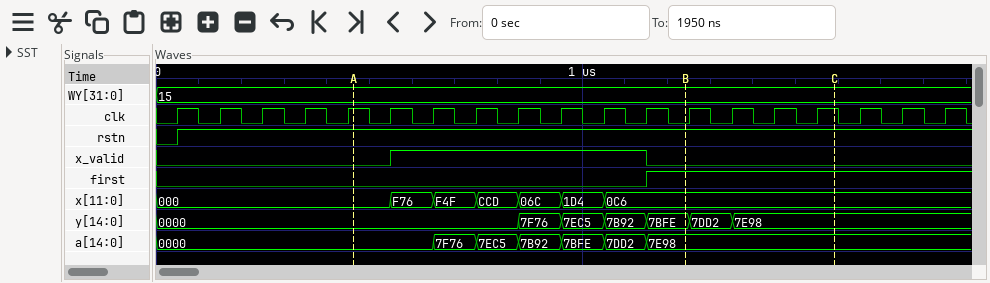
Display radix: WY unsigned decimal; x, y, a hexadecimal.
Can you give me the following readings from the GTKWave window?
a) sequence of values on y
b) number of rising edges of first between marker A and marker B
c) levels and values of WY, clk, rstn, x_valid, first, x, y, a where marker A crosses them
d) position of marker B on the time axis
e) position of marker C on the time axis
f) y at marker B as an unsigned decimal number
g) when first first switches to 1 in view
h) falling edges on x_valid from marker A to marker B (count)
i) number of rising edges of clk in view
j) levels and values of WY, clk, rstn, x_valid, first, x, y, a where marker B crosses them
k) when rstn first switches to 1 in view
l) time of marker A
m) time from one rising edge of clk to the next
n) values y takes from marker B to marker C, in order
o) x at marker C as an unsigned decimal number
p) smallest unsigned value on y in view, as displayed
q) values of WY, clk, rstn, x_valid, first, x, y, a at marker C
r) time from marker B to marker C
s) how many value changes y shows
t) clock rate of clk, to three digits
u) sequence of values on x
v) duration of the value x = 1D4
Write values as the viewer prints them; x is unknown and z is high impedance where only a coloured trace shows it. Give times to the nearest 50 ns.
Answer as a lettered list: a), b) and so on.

a) 0000, 7F76, 7EC5, 7B92, 7BFE, 7DD2, 7E98
b) 1
c) WY=15, clk=1, rstn=1, x_valid=0, first=0, x=000, y=0000, a=0000
d) 1250 ns
e) 1600 ns
f) 31742
g) 1150 ns
h) 1
i) 19
j) WY=15, clk=0, rstn=1, x_valid=0, first=1, x=0C6, y=7BFE, a=7E98
k) 50 ns
l) 450 ns
m) 100 ns
n) 7BFE, 7DD2, 7E98
o) 198
p) 0000
q) WY=15, clk=1, rstn=1, x_valid=0, first=1, x=0C6, y=7E98, a=7E98
r) 350 ns
s) 6
t) 10.0 MHz
u) 000, F76, F4F, CCD, 06C, 1D4, 0C6
v) 100 ns
